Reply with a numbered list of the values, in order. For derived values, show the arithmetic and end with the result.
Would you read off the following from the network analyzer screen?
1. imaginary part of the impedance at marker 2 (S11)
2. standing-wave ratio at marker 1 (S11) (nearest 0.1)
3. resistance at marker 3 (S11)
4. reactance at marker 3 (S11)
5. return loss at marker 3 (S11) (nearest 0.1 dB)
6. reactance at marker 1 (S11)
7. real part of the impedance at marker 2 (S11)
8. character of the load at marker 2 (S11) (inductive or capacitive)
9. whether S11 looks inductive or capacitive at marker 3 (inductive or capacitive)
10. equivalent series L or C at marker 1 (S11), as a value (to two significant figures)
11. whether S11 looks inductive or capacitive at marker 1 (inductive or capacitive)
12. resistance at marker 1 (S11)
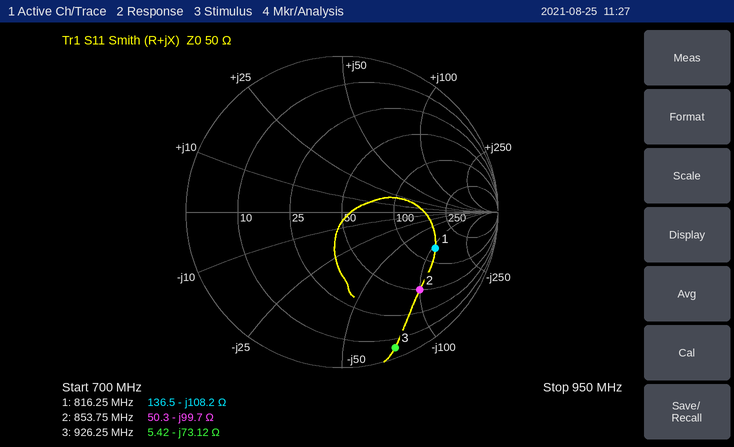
1. -99.7 Ω
2. 4.6
3. 5.42 Ω
4. -73.12 Ω
5. 0.6 dB
6. -108.2 Ω
7. 50.3 Ω
8. capacitive
9. capacitive
10. C = 1/(2π × 816.25 MHz × 108.2 Ω) ≈ 1.8 pF
11. capacitive
12. 136.5 Ω
